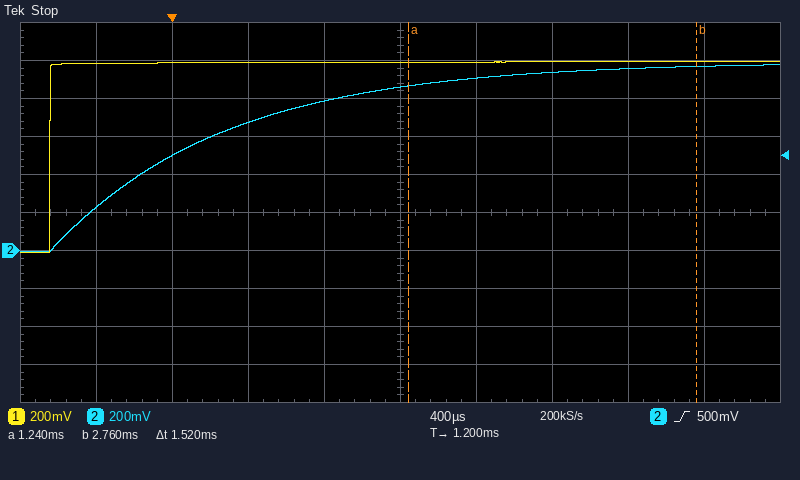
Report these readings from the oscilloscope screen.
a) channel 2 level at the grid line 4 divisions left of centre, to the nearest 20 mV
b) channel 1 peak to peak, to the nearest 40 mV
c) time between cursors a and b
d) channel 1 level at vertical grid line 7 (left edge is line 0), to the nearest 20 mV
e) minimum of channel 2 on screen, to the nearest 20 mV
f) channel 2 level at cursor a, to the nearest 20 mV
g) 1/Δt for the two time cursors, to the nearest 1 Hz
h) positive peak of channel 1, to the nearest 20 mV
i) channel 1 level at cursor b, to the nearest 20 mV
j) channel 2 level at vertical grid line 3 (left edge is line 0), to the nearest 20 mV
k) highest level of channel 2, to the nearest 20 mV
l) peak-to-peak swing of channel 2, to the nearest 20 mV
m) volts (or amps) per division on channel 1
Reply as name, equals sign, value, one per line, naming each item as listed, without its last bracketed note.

channel 2 level at the grid line 4 divisions left of centre, to the nearest 20 mV = 220 mV
channel 1 peak to peak, to the nearest 40 mV = 1.00 V
time between cursors a and b = 1.52 ms
channel 1 level at vertical grid line 7 (left edge is line 0), to the nearest 20 mV = 1.00 V
minimum of channel 2 on screen, to the nearest 20 mV = 0 mV
channel 2 level at cursor a, to the nearest 20 mV = 860 mV
1/Δt for the two time cursors, to the nearest 1 Hz = 658 Hz
positive peak of channel 1, to the nearest 20 mV = 1.00 V
channel 1 level at cursor b, to the nearest 20 mV = 1.00 V
channel 2 level at vertical grid line 3 (left edge is line 0), to the nearest 20 mV = 680 mV
highest level of channel 2, to the nearest 20 mV = 980 mV
peak-to-peak swing of channel 2, to the nearest 20 mV = 980 mV
volts (or amps) per division on channel 1 = 200 mV
